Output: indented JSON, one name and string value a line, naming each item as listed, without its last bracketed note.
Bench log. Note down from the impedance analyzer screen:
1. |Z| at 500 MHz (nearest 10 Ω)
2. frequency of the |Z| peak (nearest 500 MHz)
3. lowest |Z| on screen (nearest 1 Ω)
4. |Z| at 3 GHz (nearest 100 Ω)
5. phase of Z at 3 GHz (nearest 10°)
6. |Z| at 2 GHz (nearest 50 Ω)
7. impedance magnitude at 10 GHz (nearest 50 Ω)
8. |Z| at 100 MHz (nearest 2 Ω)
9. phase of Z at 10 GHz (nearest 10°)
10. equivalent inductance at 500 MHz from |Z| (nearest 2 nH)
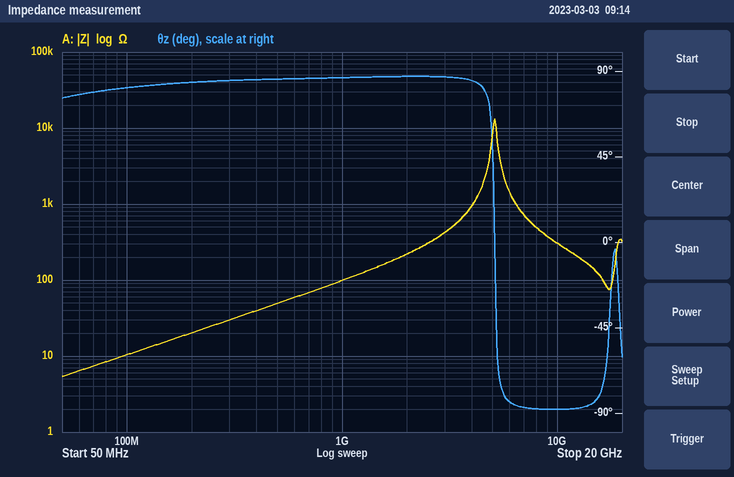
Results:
{
  "|Z| at 500 MHz": "50 Ω",
  "frequency of the |Z| peak": "5.0 GHz",
  "lowest |Z| on screen": "5 Ω",
  "|Z| at 3 GHz": "400 Ω",
  "phase of Z at 3 GHz": "90°",
  "|Z| at 2 GHz": "200 Ω",
  "impedance magnitude at 10 GHz": "300 Ω",
  "|Z| at 100 MHz": "10 Ω",
  "phase of Z at 10 GHz": "-90°",
  "equivalent inductance at 500 MHz from |Z|": "16 nH"
}
